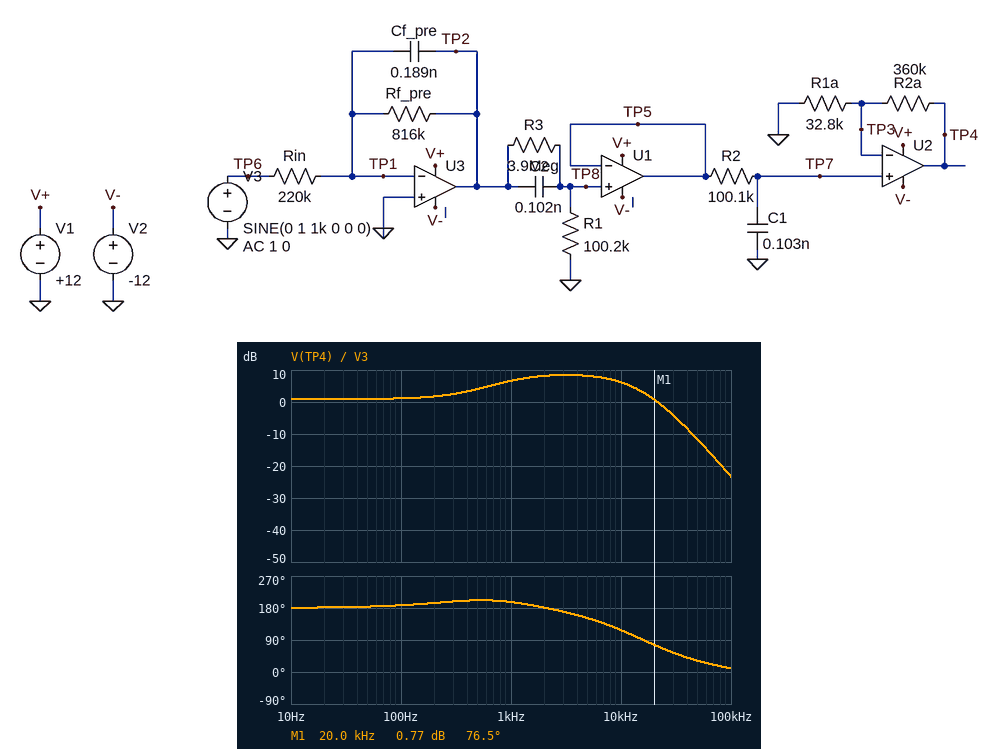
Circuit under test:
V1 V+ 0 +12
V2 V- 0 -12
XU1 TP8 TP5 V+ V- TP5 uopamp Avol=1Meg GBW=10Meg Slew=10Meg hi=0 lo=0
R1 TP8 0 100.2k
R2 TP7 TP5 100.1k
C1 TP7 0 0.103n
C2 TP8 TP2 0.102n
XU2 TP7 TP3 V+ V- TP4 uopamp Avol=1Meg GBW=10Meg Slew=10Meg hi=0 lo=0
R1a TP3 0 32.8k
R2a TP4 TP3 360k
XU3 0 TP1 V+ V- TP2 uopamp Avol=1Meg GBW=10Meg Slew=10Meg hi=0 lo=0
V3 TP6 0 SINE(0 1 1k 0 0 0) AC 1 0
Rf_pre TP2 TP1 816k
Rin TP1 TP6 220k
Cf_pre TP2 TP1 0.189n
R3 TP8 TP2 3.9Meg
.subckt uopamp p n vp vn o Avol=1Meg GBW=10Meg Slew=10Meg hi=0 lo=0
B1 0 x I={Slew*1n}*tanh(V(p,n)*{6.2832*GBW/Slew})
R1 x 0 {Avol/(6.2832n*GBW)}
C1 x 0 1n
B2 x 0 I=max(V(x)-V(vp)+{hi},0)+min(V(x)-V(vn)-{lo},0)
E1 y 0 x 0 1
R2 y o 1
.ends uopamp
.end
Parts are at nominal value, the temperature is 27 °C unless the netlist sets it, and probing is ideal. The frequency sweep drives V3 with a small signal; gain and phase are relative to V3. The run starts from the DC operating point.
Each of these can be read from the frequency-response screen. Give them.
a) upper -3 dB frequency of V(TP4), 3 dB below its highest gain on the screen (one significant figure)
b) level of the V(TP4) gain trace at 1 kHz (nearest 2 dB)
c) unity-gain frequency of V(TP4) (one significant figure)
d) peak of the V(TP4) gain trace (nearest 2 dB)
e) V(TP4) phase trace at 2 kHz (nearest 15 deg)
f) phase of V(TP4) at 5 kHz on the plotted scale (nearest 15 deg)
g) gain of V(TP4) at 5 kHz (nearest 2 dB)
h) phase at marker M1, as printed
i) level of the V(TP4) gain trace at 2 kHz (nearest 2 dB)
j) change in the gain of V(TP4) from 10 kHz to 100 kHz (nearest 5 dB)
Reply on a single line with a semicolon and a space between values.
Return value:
10 kHz; 6 dB; 20 kHz; 8 dB; 180 deg; 150 deg; 8 dB; 76.5 deg; 8 dB; -30 dB
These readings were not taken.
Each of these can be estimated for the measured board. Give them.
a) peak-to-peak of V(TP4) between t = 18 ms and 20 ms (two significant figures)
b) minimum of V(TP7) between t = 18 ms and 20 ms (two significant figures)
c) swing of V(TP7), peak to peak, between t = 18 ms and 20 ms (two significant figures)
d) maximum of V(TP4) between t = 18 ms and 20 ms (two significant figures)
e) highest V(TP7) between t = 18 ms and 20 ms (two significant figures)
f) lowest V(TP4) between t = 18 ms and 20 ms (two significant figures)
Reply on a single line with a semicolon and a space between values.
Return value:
4.3 V; -180 mV; 360 mV; 2.1 V; 180 mV; -2.1 V
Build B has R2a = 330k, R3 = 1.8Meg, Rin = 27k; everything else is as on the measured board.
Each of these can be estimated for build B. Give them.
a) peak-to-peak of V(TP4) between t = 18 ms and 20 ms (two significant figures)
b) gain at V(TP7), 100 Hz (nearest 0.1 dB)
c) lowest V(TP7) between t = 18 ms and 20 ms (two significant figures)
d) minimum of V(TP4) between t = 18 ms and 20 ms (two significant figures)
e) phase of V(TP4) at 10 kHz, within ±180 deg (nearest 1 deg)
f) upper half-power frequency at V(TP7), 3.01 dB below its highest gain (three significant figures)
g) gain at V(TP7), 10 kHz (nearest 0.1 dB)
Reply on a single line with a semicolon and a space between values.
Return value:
24 V; 4.1 dB; -1.6 V; -12 V; 116 deg; 11.0 kHz; 2.6 dB
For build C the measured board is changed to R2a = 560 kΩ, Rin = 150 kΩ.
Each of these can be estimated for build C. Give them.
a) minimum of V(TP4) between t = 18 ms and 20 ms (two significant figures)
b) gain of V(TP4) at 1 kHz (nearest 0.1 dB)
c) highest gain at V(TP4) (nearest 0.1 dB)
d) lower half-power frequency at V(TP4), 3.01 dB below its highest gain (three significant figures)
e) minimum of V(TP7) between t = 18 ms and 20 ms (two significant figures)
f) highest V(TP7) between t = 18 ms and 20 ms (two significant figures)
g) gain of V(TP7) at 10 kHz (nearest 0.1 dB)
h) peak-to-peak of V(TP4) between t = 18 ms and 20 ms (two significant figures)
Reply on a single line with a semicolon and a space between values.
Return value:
-4.7 V; 13.5 dB; 15.3 dB; 714 Hz; -260 mV; 260 mV; -12.1 dB; 9.5 V
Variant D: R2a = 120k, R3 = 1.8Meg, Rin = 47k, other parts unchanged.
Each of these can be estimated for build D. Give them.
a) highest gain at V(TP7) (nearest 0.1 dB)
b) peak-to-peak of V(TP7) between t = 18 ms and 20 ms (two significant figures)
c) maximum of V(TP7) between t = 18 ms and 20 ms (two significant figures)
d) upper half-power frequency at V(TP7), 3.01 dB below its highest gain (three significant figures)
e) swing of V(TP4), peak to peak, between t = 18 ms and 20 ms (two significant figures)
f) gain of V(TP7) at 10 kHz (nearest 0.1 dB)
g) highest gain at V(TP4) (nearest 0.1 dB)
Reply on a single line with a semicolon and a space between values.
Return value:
0.3 dB; 2.0 V; 1.0 V; 11.0 kHz; 9.3 V; -2.2 dB; 13.7 dB
